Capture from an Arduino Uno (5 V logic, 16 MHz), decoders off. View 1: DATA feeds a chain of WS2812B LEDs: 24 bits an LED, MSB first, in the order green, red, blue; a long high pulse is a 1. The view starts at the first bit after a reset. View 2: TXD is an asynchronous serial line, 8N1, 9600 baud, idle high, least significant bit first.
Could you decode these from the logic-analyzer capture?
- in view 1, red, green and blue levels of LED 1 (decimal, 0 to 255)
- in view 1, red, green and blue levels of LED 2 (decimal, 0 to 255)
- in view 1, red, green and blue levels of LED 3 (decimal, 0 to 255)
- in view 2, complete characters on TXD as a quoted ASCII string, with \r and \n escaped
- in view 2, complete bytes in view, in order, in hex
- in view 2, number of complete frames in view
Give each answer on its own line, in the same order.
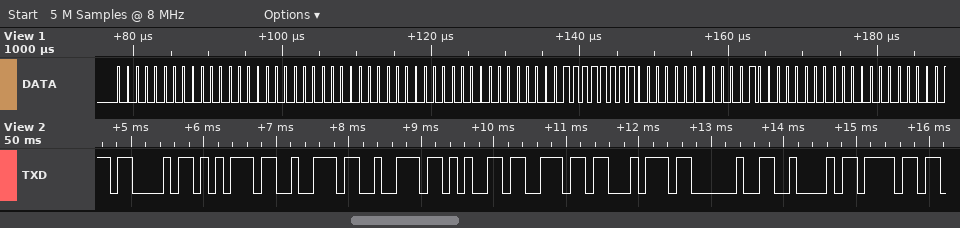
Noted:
0, 0, 0
0, 0, 0
0, 255, 8
"Current Bo"
43 75 72 72 65 6E 74 20 42 6F
10
